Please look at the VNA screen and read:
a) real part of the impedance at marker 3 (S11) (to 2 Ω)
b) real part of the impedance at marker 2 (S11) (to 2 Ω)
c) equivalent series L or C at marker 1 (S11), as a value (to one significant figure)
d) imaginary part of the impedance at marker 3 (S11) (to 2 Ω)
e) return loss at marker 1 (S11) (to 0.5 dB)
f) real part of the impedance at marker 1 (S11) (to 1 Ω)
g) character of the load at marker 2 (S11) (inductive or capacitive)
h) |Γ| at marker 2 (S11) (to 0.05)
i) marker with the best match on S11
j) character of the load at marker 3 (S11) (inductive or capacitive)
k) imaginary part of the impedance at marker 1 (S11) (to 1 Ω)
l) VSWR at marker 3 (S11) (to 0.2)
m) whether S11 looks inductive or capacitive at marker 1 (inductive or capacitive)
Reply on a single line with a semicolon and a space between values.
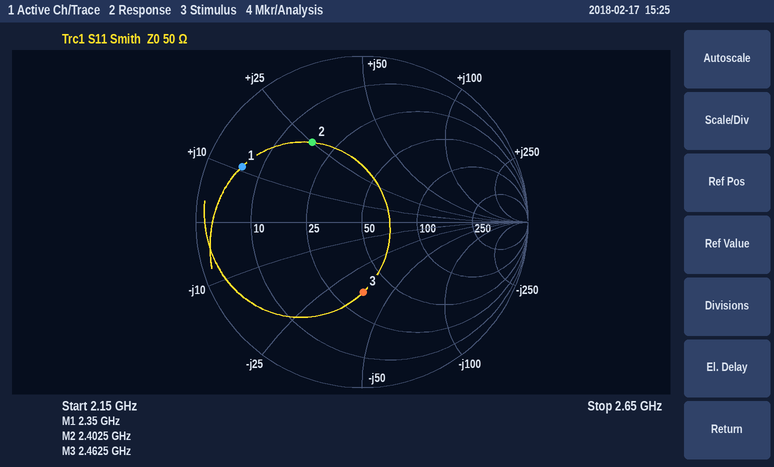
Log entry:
36 Ω; 18 Ω; 700 pH; -36 Ω; 2.0 dB; 6 Ω; inductive; 0.55; marker 3; capacitive; +11 Ω; 2.4; inductive
